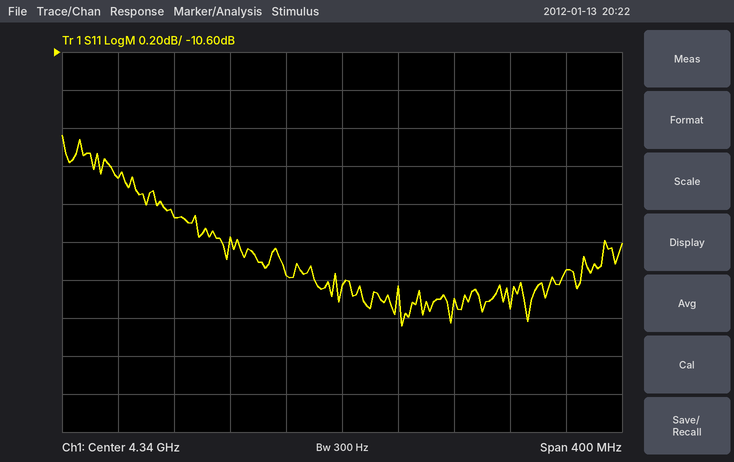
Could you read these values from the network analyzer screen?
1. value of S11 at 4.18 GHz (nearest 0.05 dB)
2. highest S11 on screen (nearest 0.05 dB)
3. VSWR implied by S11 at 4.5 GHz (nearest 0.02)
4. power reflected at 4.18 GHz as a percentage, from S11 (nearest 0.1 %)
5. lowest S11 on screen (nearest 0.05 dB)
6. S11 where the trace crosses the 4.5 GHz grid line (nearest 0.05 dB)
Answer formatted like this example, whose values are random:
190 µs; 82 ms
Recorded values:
-11.25 dB; -11.05 dB; 1.70; 7.5 %; -12.05 dB; -11.75 dB
